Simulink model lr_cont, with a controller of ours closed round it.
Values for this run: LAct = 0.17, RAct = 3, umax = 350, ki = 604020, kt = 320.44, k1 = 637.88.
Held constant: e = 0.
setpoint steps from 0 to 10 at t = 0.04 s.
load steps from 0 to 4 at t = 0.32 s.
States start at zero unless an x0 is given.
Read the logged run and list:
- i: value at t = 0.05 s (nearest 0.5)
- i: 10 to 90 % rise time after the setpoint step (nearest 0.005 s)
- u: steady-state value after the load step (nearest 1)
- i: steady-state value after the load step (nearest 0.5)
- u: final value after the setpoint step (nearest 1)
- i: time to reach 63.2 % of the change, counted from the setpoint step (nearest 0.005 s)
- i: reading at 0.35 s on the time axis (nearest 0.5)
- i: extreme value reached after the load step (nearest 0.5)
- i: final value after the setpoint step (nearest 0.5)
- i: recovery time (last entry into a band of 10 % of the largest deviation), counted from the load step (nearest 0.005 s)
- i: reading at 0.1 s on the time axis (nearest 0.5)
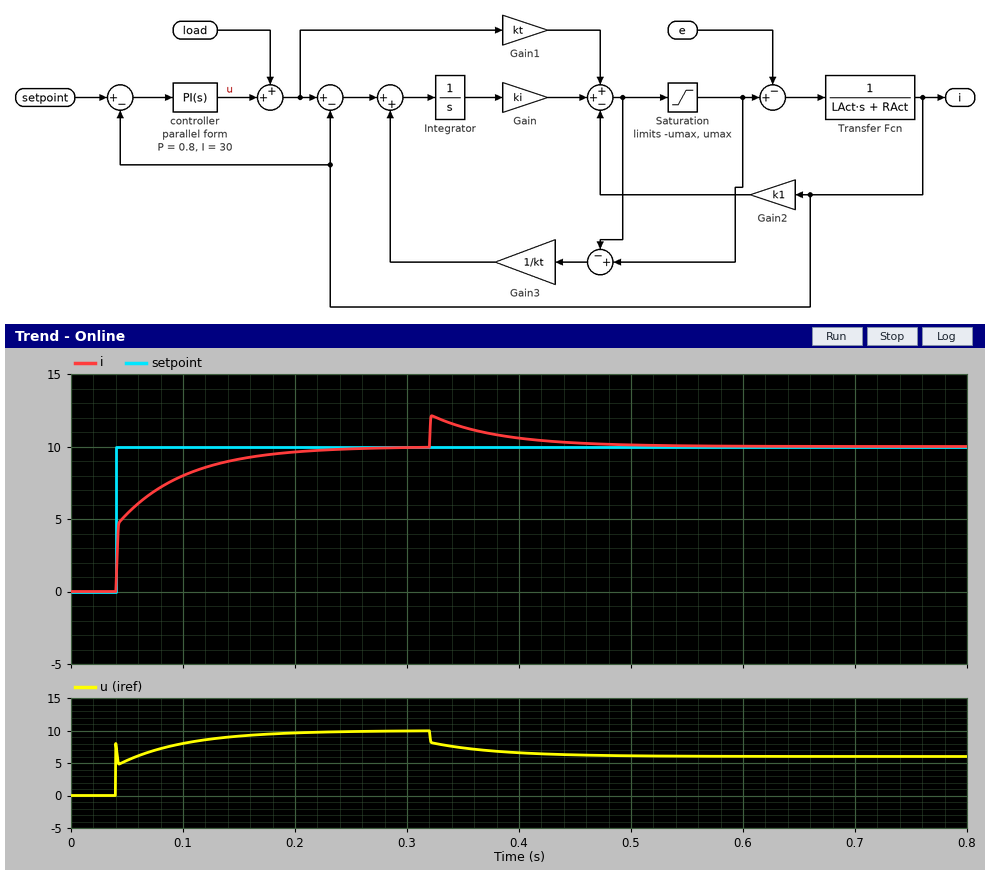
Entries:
5.5
0.100 s
6
10.0
10
0.025 s
11.5
12.0
10.0
0.140 s
8.0
